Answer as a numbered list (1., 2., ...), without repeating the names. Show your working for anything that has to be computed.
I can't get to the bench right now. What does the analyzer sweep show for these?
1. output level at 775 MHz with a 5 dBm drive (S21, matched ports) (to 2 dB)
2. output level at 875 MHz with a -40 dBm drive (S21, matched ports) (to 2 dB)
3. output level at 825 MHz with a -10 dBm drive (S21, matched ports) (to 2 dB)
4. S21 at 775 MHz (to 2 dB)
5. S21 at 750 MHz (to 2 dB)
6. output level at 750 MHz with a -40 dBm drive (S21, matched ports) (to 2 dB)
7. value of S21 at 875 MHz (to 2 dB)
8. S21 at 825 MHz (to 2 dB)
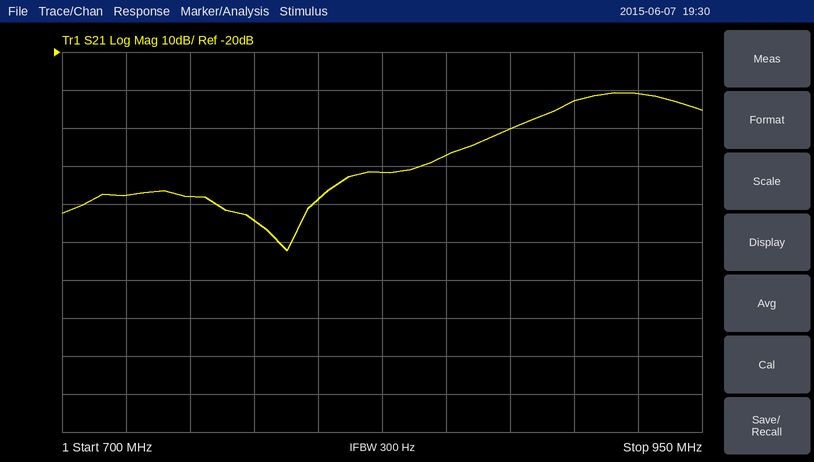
1. 5 dBm + (-64 dB) = -60 dBm
2. -40 dBm + (-40 dB) = -80 dBm
3. -10 dBm + (-52 dB) = -62 dBm
4. -64 dB
5. -58 dB
6. -40 dBm + (-58 dB) = -98 dBm
7. -40 dB
8. -52 dB
